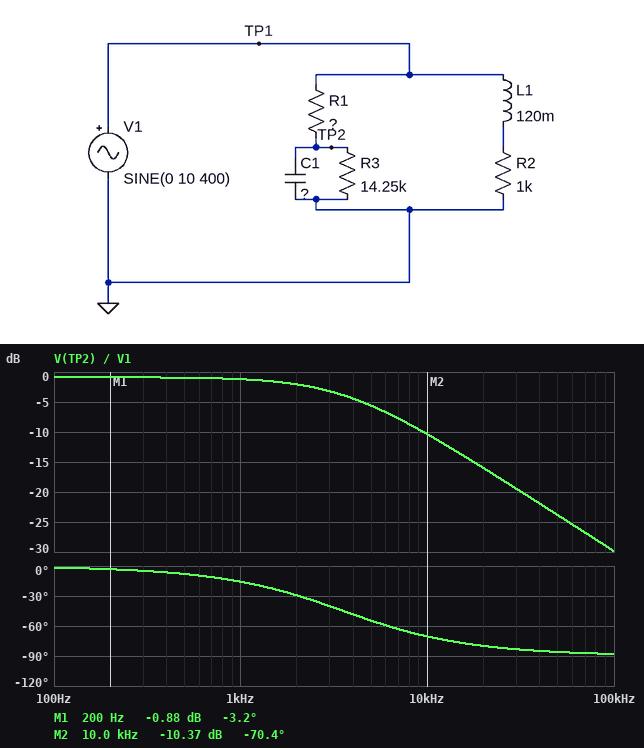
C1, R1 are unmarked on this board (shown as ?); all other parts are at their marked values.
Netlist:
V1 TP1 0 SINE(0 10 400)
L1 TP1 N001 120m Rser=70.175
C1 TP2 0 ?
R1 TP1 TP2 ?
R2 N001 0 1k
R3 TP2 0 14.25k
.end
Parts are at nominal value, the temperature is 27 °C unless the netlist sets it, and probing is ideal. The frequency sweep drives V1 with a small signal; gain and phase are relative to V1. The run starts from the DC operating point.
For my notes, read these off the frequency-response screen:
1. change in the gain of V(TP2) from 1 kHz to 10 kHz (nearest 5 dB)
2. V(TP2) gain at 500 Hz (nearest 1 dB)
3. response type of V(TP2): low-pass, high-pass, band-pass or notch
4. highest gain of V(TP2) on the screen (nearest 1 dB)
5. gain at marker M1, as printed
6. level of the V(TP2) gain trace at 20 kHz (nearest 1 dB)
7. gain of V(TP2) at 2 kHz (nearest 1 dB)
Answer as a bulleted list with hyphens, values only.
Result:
- -10 dB
- -1 dB
- low-pass
- -1 dB
- -0.88 dB
- -16 dB
- -2 dB
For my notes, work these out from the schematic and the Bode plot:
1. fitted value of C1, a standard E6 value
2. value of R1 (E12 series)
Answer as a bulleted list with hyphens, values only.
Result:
- 33 nF
- 1.5 kΩ
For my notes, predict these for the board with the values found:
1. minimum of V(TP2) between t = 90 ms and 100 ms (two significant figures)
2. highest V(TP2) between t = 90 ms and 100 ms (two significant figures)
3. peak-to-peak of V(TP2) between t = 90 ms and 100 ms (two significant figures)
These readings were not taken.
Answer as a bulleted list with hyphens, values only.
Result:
- -9.0 V
- 9.0 V
- 18 V
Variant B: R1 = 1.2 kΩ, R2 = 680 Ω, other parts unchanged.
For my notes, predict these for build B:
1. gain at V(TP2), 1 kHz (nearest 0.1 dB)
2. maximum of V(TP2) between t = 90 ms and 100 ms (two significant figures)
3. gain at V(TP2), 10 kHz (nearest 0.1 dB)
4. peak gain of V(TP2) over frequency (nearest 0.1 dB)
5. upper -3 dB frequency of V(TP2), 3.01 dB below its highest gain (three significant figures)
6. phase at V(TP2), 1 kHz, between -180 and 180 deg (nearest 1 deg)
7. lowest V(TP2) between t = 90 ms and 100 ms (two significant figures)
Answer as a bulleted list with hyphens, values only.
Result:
- -0.9 dB
- 9.2 V
- -8.7 dB
- -0.7 dB
- 4.36 kHz
- -13 deg
- -9.2 V
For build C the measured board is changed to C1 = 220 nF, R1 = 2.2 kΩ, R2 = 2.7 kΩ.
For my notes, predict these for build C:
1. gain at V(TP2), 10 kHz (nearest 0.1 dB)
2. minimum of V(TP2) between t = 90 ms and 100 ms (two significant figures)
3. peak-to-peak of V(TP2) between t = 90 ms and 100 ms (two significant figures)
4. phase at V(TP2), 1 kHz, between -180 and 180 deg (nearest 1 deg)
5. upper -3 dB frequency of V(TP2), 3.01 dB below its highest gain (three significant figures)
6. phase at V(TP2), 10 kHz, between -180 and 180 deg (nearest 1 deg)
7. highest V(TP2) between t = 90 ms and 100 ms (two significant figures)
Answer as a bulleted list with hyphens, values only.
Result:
- -29.7 dB
- -6.0 V
- 12 V
- -69 deg
- 380 Hz
- -88 deg
- 6.0 V
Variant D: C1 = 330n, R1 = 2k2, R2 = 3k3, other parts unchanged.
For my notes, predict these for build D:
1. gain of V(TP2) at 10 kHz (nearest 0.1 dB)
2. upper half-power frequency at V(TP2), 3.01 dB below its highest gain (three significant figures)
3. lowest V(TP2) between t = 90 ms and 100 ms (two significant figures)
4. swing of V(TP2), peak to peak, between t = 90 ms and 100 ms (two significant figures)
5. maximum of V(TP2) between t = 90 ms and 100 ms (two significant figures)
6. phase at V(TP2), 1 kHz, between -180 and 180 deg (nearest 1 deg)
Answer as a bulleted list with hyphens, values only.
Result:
- -33.2 dB
- 253 Hz
- -4.6 V
- 9.3 V
- 4.6 V
- -76 deg
